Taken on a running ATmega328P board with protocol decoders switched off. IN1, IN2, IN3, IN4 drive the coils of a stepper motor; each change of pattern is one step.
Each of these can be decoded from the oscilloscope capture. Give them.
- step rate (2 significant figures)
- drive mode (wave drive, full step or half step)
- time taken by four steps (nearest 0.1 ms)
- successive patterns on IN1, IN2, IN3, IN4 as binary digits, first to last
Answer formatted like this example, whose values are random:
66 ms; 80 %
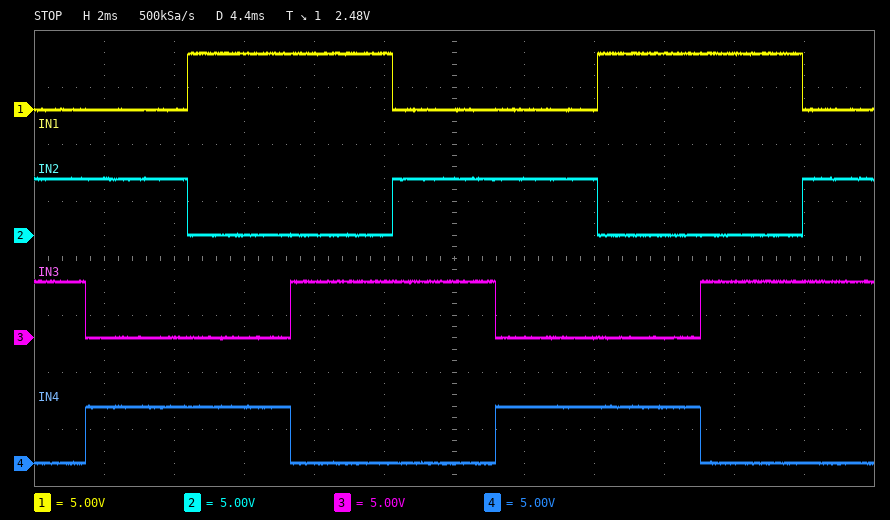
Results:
340 steps/s; full step; 11.7 ms; 0110 0101 1001 1010 0110 0101 1001 1010 0110
